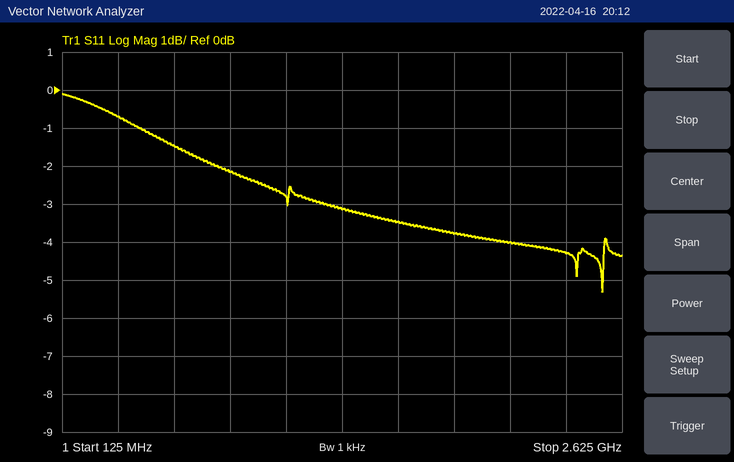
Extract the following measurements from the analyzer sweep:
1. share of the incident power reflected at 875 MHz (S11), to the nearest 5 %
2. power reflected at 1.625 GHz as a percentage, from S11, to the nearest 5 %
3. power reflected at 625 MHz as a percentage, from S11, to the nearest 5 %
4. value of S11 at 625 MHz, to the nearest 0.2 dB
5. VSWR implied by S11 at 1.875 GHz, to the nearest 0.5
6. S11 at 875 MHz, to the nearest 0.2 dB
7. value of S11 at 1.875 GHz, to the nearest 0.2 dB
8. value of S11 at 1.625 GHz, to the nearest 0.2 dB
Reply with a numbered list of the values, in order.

1. 60 %
2. 45 %
3. 70 %
4. -1.4 dB
5. 4.5
6. -2.2 dB
7. -3.8 dB
8. -3.4 dB
